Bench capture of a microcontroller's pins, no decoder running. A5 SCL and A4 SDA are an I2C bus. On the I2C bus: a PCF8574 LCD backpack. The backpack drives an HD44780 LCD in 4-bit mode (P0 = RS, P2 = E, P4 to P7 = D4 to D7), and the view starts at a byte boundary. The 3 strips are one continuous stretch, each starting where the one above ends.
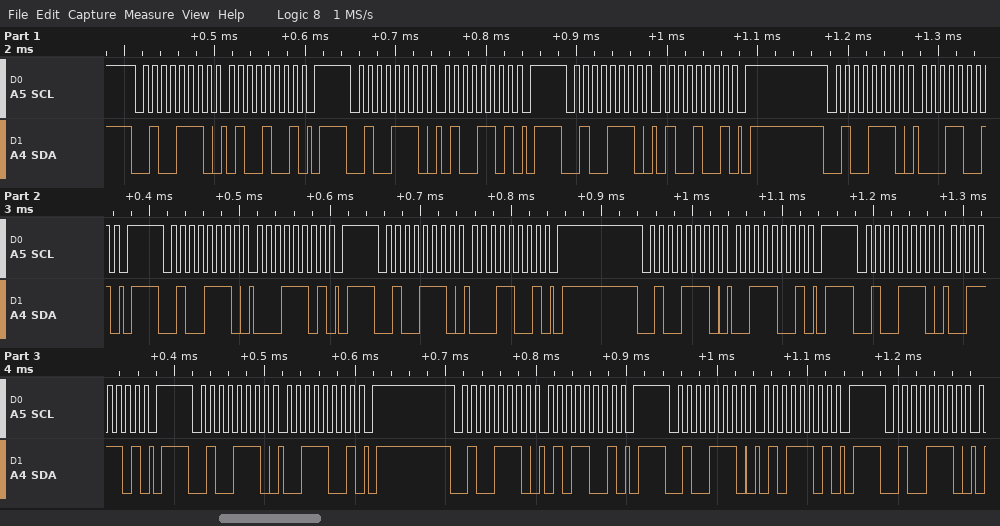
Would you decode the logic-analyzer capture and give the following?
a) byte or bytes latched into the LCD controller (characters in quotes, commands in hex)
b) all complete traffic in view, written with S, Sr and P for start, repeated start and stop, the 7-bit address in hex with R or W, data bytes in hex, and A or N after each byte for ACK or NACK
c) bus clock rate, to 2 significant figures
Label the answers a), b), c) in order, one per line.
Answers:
a) 'A'
b) S 27W A 49 A P S 27W A 4D A P S 27W A 49 A P S 27W A 19 A P S 27W A 1D A P S 27W A 19 A P S 27W A 39 A P S 27W A 3D A P S 27W A 39 A P S 27W A 59 A P S 27W A 5D A P S 27W A
c) 100 kHz
